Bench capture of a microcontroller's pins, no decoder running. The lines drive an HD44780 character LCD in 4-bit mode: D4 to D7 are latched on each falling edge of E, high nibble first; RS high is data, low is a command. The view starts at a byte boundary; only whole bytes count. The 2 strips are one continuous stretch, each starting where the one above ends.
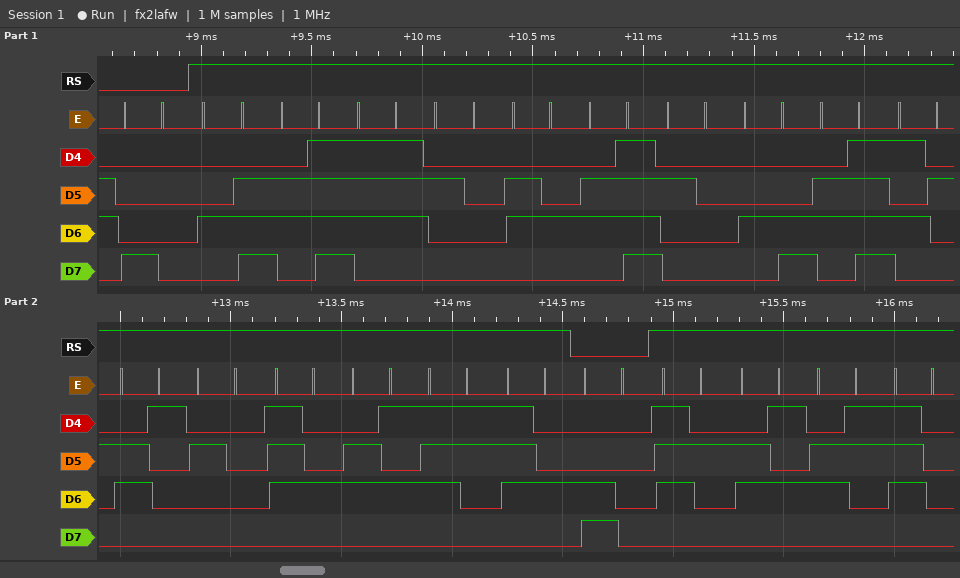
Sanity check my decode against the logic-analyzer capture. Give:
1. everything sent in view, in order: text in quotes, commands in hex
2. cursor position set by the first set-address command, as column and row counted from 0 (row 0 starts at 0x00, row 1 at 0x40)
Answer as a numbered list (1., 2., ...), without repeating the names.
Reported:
1. 0x80 "Now do LoRa test" 0xC0 "recp"
2. column 0, row 0
